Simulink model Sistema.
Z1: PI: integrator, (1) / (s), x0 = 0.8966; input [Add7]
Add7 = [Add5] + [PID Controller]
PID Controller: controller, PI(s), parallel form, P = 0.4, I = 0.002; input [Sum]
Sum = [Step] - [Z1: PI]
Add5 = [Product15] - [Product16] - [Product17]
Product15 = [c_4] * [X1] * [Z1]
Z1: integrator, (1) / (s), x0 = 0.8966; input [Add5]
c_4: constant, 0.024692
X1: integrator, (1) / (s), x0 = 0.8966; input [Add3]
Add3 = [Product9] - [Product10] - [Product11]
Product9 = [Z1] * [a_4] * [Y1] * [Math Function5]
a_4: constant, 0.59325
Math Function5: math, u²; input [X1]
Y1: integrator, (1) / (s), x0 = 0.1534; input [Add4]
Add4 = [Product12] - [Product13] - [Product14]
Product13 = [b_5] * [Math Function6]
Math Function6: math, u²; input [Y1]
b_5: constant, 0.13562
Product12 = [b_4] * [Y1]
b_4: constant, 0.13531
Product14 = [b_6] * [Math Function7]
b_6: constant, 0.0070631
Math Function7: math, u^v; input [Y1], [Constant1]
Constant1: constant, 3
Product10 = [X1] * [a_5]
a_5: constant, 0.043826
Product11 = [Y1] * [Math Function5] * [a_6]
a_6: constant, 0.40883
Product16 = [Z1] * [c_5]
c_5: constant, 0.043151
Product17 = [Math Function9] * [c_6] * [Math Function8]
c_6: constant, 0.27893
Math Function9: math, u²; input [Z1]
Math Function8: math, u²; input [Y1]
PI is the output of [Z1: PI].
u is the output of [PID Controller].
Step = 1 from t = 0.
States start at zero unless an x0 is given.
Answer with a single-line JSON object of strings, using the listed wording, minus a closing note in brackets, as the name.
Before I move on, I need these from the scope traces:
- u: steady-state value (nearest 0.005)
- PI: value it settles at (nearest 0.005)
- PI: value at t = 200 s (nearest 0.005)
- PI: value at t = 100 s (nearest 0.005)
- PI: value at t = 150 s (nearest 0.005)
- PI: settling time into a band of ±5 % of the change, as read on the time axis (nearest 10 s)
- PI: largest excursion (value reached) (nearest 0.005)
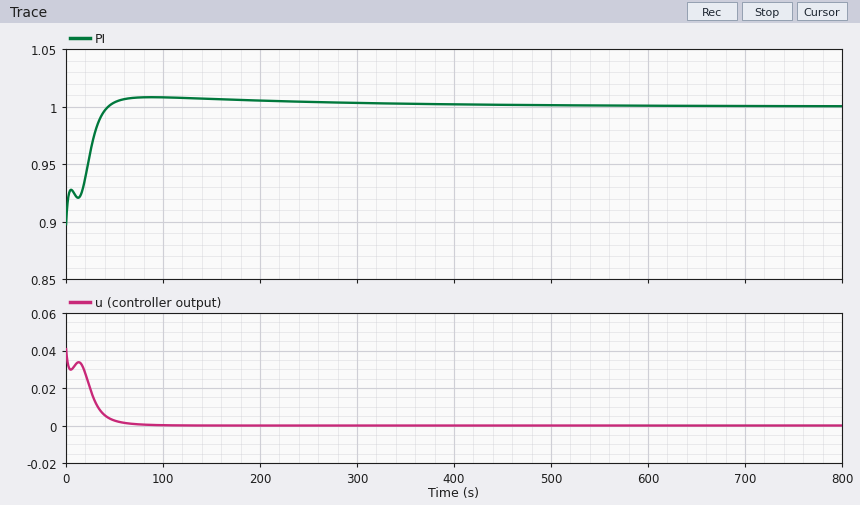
{"u: steady-state value": "0.000", "PI: value it settles at": "1.000", "PI: value at t = 200 s": "1.005", "PI: value at t = 100 s": "1.010", "PI: value at t = 150 s": "1.005", "PI: settling time into a band of ±5 % of the change, as read on the time axis": "200 s", "PI: largest excursion (value reached)": "1.010"}
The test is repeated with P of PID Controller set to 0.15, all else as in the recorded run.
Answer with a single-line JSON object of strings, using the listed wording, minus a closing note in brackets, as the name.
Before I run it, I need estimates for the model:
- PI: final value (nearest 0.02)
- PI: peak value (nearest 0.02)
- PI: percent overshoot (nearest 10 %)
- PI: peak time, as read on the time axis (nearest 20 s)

{"PI: final value": "1.00", "PI: peak value": "1.04", "PI: percent overshoot": "40 %", "PI: peak time, as read on the time axis": "60 s"}
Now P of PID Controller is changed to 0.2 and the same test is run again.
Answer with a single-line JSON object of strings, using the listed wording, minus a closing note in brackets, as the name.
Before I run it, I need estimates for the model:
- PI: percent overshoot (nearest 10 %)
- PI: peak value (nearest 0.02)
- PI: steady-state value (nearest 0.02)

{"PI: percent overshoot": "30 %", "PI: peak value": "1.02", "PI: steady-state value": "1.00"}
